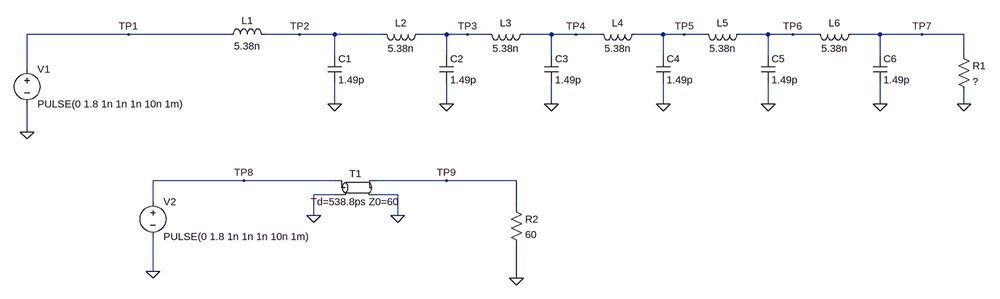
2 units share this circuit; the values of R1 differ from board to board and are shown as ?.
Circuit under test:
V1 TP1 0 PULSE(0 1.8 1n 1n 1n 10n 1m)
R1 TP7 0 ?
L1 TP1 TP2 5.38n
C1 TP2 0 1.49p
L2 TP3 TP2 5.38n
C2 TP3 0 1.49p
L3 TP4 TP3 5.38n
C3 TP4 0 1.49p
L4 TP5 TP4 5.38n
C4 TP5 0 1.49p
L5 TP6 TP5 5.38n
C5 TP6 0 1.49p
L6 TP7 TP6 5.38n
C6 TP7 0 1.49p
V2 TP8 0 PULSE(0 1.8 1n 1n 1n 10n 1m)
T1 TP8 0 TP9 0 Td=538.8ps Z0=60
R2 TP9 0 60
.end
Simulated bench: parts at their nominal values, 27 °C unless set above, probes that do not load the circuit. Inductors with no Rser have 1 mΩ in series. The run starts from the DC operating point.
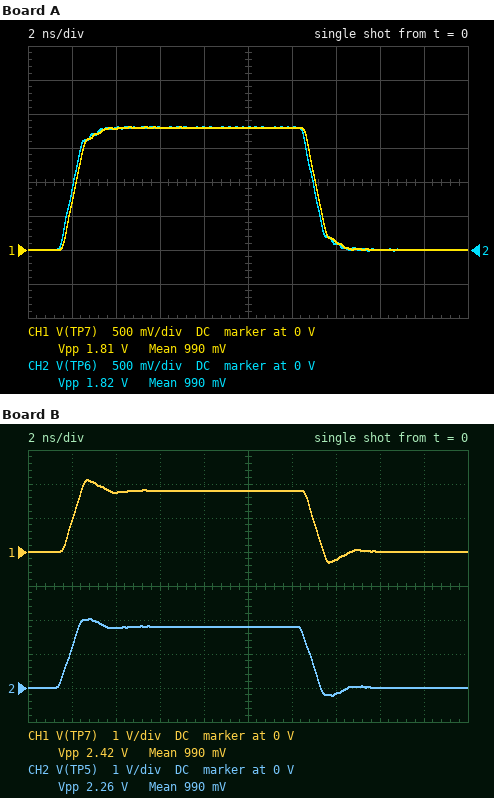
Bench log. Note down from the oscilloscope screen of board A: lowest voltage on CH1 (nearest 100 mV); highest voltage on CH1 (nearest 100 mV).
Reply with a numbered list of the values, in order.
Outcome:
1. 0 V
2. 1.8 V
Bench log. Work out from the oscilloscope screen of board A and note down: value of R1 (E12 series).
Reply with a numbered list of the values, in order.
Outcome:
1. 47 Ω
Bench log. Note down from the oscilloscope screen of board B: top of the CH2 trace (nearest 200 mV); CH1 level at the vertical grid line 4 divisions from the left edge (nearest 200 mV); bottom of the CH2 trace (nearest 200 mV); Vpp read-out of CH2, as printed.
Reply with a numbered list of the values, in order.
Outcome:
1. 2.0 V
2. 1.8 V
3. -200 mV
4. 2.26 V
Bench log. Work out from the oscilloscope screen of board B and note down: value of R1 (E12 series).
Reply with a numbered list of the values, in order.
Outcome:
1. 82 Ω
